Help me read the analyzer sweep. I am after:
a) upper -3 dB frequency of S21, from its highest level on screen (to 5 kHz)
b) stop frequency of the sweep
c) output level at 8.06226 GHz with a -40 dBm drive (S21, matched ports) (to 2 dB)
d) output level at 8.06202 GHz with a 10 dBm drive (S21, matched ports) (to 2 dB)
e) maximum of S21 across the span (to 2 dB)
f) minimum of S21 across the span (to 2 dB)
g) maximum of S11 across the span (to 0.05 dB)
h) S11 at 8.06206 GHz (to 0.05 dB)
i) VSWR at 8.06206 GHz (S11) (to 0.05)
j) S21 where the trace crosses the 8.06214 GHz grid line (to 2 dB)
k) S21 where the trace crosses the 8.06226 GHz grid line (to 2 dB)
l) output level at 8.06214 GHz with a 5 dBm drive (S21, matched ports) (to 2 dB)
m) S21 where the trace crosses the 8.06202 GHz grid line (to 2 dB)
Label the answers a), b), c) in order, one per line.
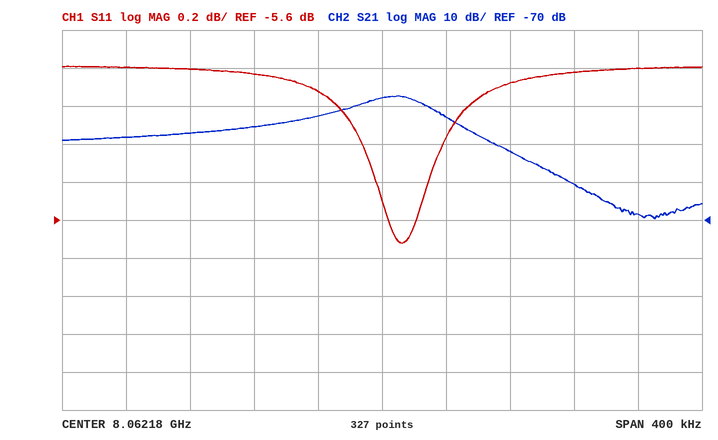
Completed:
a) 8.062210 GHz
b) 8.06238 GHz
c) -92 dBm
d) -38 dBm
e) -38 dB
f) -70 dB
g) -4.80 dB
h) -4.80 dB
i) 3.70
j) -42 dB
k) -52 dB
l) -38 dBm
m) -48 dB
